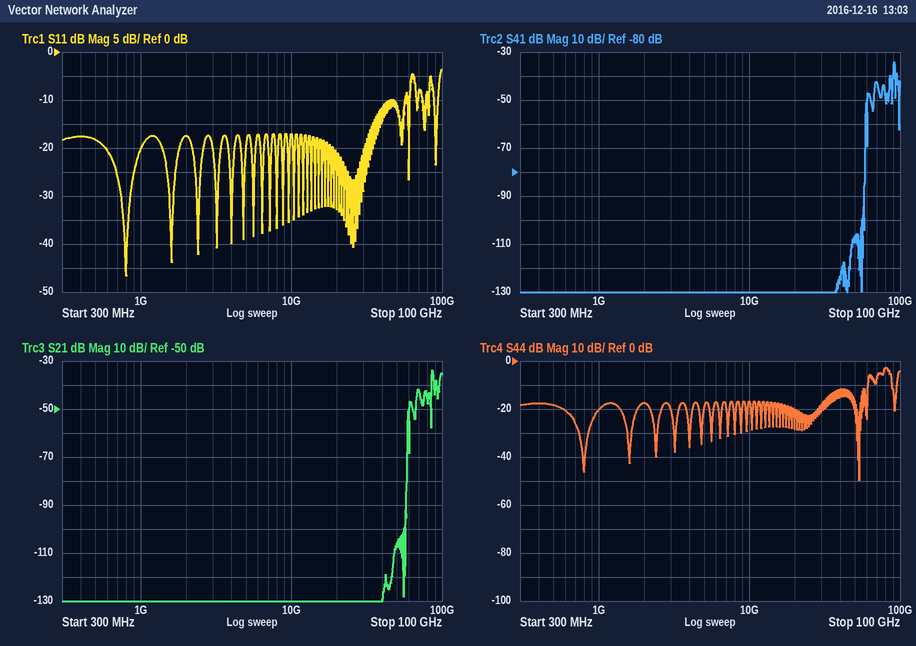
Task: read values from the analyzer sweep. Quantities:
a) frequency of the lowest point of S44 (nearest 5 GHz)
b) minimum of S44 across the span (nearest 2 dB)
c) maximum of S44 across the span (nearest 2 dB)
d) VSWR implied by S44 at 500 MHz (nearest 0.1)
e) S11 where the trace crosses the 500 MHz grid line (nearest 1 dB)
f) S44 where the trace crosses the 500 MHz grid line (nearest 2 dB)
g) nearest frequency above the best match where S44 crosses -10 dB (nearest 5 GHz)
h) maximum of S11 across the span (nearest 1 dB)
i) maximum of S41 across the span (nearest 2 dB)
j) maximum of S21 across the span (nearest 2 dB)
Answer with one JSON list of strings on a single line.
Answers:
["55 GHz", "-50 dB", "-2 dB", "1.3", "-18 dB", "-18 dB", "60 GHz", "-4 dB", "-34 dB", "-34 dB"]
